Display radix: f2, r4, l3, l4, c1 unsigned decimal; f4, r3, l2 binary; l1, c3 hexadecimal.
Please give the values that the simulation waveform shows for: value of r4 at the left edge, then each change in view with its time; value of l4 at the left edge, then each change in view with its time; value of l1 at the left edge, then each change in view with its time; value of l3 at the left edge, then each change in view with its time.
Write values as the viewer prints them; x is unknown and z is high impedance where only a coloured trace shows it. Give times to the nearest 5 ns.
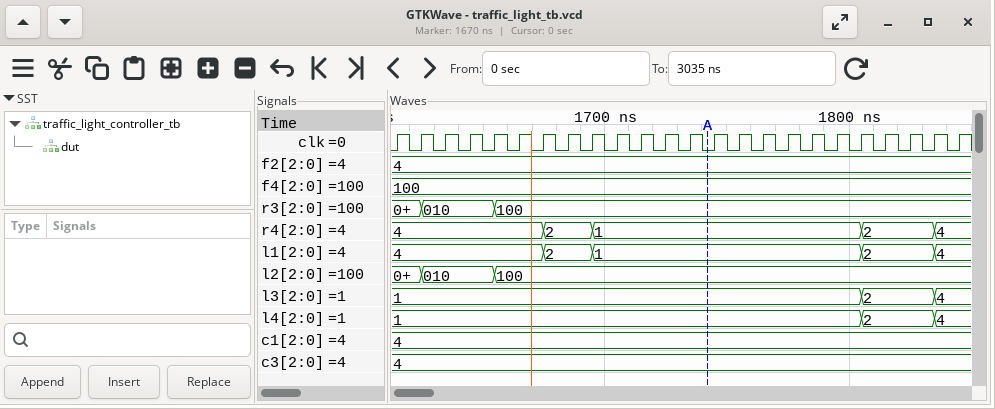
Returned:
4, 2 at 1675 ns, 1 at 1695 ns, 2 at 1805 ns, 4 at 1835 ns
1, 2 at 1805 ns, 4 at 1835 ns
4, 2 at 1675 ns, 1 at 1695 ns, 2 at 1805 ns, 4 at 1835 ns
1, 2 at 1805 ns, 4 at 1835 ns
